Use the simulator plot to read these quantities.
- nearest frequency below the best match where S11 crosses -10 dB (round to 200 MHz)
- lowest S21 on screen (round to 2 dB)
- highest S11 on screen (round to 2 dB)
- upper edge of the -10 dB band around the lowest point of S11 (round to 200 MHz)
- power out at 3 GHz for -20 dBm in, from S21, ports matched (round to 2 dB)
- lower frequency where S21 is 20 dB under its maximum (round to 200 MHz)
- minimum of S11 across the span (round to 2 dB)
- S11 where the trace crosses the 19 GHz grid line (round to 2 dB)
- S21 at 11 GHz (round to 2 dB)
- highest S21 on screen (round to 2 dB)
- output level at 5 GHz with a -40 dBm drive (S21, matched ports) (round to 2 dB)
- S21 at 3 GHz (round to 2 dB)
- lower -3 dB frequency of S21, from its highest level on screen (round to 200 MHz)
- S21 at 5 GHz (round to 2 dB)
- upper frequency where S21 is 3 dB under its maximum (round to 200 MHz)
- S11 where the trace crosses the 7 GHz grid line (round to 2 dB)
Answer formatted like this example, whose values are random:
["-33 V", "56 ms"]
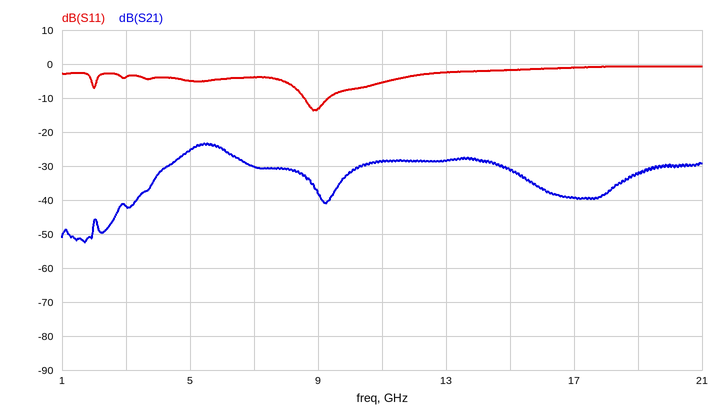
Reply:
["8.6 GHz", "-52 dB", "0 dB", "9.4 GHz", "-62 dBm", "2.8 GHz", "-14 dB", "0 dB", "-28 dB", "-24 dB", "-66 dBm", "-42 dB", "4.8 GHz", "-26 dB", "6.2 GHz", "-4 dB"]
